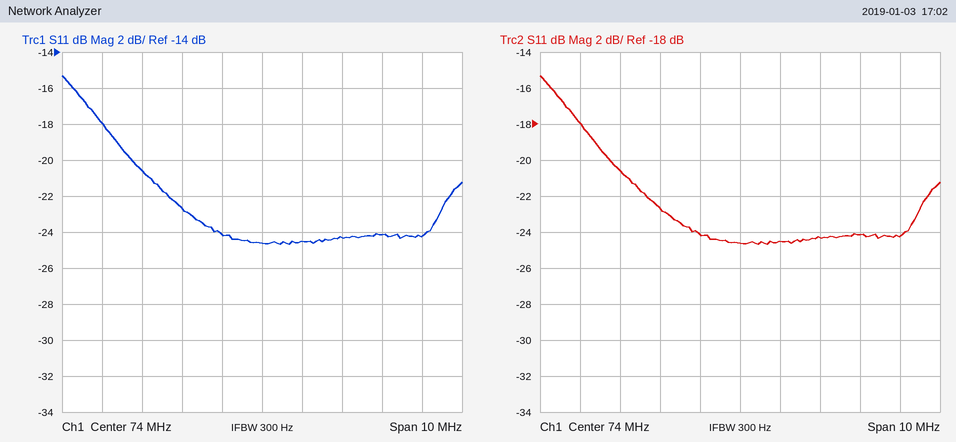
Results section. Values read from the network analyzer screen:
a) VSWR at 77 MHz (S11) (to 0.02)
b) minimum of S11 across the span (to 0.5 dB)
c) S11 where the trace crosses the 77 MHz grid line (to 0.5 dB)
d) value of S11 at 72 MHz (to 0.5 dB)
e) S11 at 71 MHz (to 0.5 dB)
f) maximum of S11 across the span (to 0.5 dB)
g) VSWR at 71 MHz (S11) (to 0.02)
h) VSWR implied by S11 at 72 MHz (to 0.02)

1.14
-24.5 dB
-24.0 dB
-22.5 dB
-20.5 dB
-15.5 dB
1.20
1.16
